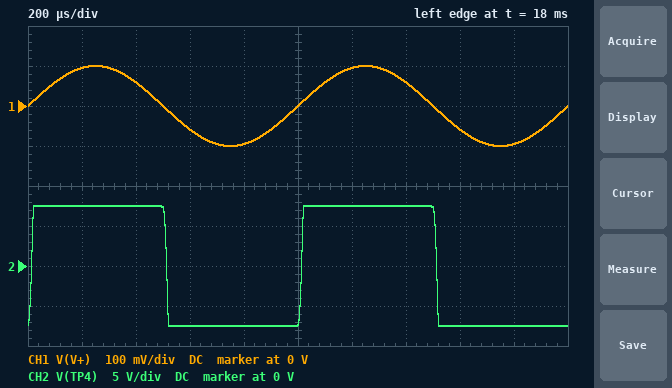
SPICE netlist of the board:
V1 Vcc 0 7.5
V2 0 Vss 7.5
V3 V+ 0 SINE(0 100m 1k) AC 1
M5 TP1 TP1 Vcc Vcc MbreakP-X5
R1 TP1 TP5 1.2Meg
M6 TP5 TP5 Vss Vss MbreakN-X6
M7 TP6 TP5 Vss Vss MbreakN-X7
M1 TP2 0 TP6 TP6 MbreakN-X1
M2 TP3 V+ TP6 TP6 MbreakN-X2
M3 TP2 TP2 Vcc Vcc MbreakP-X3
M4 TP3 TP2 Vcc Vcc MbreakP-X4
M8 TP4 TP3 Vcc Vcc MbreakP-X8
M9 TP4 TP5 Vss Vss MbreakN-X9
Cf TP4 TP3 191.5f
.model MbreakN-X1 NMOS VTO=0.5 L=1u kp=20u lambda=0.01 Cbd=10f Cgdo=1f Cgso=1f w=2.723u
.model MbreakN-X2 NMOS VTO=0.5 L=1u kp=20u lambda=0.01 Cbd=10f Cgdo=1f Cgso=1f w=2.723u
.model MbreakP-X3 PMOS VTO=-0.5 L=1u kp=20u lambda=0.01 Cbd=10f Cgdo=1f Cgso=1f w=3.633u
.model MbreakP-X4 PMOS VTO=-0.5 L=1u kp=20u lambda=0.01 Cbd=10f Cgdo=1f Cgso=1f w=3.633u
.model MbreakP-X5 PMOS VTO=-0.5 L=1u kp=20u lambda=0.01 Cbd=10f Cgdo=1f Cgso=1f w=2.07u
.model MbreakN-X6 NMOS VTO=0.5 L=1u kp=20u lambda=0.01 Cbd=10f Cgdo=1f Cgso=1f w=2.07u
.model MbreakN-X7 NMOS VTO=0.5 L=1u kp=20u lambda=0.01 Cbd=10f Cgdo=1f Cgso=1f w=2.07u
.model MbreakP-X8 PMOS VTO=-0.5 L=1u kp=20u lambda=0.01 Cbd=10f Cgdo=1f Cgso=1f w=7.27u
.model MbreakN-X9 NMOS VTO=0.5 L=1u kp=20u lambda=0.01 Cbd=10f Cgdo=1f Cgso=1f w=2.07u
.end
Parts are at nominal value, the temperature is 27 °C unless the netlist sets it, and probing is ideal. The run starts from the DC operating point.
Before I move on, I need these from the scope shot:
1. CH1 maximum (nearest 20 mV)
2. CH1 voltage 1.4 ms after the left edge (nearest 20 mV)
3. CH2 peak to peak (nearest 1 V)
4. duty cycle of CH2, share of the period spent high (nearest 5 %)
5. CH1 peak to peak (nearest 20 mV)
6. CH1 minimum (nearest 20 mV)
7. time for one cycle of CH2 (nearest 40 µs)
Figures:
100 mV
60 mV
15 V
50 %
200 mV
-100 mV
1.00 ms
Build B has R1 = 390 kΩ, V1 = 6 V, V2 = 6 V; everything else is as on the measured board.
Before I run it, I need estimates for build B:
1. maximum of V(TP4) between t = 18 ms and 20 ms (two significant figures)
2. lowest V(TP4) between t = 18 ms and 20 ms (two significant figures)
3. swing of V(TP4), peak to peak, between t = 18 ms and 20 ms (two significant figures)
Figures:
6.0 V
-6.0 V
12 V
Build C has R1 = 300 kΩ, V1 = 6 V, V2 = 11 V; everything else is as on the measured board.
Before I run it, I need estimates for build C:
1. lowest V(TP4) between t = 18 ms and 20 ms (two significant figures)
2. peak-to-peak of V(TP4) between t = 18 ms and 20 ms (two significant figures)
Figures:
-11 V
17 V
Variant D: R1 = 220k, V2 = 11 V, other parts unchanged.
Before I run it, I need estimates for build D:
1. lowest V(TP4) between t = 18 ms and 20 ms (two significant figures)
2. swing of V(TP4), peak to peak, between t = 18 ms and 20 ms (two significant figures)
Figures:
-11 V
18 V
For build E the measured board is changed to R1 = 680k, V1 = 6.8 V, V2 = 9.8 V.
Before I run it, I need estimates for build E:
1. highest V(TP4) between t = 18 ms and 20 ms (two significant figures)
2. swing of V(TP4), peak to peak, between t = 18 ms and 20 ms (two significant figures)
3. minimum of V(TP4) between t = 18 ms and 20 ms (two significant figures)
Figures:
6.8 V
17 V
-9.8 V
